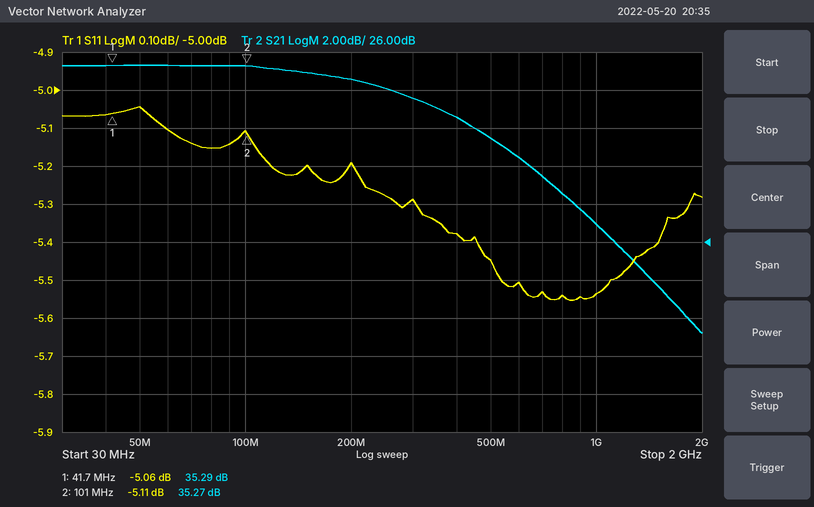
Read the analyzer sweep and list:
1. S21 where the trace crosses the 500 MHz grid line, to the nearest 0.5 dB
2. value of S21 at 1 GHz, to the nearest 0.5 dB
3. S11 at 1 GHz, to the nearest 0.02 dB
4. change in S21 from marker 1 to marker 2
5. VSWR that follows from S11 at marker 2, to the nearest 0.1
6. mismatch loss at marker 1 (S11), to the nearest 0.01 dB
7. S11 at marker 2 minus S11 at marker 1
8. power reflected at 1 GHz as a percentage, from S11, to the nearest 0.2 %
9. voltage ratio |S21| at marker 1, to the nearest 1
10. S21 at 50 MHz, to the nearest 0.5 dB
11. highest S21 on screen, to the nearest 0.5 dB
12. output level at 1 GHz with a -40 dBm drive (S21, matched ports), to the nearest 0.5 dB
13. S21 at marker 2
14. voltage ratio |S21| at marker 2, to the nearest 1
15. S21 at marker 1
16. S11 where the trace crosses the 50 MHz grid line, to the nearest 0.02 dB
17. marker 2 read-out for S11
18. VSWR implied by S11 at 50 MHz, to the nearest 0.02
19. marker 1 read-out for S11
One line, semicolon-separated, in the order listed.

31.5 dB; 27.0 dB; -5.54 dB; -0.02 dB; 3.5; 1.62 dB; -0.05 dB; 28.0 %; 58; 35.5 dB; 35.5 dB; -13.0 dBm; 35.27 dB; 58; 35.29 dB; -5.04 dB; -5.11 dB; 3.54; -5.06 dB
